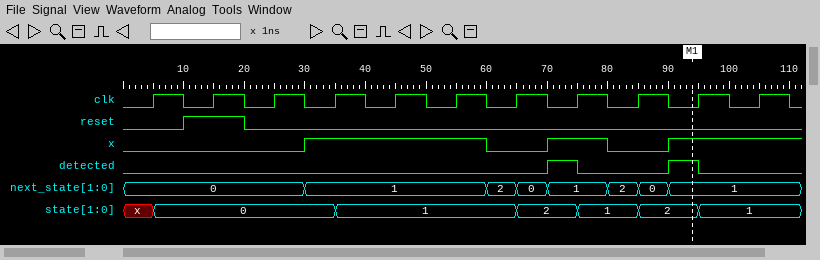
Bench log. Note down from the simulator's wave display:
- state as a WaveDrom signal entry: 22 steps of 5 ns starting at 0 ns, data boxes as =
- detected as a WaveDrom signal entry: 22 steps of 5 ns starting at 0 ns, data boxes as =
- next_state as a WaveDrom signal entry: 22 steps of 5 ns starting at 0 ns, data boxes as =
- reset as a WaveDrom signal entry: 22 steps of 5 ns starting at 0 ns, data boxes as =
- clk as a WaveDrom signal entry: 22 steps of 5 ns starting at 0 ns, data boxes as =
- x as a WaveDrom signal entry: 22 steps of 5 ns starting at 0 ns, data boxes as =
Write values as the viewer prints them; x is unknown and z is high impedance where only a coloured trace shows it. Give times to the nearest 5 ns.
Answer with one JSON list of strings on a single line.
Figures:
["{name: 'state', wave: 'x=.....=.....=.=.=.=..', data: '0 1 2 1 2 1'}", "{name: 'detected', wave: '0.............10..10..'}", "{name: 'next_state', wave: '=.....=.....===.===...', data: '0 1 2 0 1 2 0 1'}", "{name: 'reset', wave: '0.1.0.................'}", "{name: 'clk', wave: '0101010101010101010101'}", "{name: 'x', wave: '0.....1.....0.1.0.1...'}"]
